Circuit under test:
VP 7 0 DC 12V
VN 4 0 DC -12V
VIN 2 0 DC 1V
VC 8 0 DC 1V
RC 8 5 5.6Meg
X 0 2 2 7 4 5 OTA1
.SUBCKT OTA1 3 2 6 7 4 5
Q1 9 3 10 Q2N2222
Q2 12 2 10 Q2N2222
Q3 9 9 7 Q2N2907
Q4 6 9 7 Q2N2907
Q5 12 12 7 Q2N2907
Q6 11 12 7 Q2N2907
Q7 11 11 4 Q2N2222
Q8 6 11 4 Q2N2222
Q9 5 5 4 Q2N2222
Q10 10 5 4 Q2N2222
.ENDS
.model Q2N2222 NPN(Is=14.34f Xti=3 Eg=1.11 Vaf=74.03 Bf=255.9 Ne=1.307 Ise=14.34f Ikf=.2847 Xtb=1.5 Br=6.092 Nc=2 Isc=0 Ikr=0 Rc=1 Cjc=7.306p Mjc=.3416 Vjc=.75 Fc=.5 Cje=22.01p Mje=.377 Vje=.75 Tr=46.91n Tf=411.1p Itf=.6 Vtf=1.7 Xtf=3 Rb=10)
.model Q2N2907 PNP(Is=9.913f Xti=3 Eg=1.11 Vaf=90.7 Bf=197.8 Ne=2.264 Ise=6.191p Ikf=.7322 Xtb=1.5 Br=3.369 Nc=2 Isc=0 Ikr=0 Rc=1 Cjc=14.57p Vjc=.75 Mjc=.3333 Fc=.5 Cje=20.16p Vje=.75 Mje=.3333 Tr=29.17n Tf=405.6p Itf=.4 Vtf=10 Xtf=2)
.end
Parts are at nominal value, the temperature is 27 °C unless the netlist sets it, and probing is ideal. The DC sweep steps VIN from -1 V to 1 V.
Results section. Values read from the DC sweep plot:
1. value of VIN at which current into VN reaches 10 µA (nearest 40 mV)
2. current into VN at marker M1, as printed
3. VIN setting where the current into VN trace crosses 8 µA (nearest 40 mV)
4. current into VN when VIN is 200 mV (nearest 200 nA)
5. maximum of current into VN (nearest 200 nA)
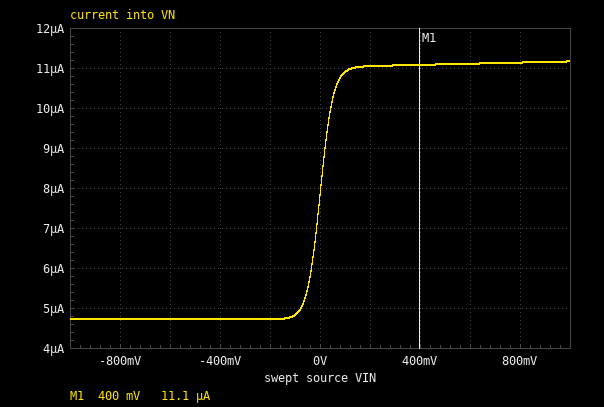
40 mV
11.1 µA
0 V
11.0 µA
11.2 µA
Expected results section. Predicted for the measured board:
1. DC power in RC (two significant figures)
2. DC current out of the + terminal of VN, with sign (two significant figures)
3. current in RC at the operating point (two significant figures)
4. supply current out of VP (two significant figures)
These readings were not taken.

28 µW
-11 µA
2.2 µA
5.5 µA
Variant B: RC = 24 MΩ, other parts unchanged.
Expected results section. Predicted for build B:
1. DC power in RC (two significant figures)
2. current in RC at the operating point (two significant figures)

6.6 µW
520 nA
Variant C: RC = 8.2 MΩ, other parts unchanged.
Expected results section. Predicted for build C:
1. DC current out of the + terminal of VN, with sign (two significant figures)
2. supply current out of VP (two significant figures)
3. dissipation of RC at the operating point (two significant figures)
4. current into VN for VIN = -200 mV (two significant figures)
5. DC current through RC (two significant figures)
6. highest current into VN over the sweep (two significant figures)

-7.6 µA
3.7 µA
19 µW
3.2 µA
1.5 µA
7.6 µA
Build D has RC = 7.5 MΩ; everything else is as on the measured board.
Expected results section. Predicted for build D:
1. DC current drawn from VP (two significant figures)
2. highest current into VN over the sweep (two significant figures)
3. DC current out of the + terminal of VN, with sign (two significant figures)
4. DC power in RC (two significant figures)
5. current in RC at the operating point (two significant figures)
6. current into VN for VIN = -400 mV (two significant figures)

4.1 µA
8.3 µA
-8.3 µA
21 µW
1.7 µA
3.5 µA
